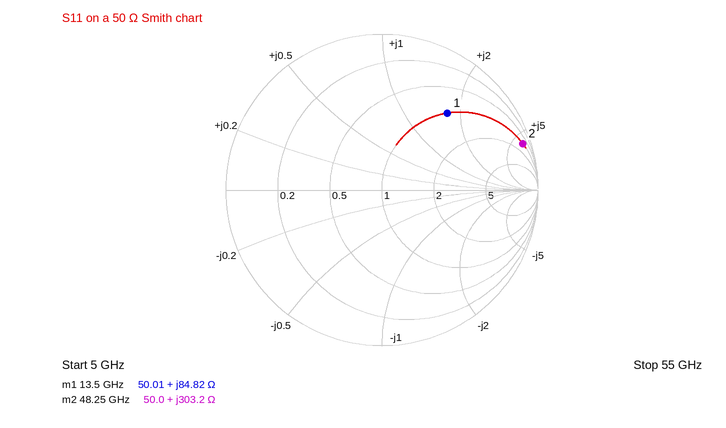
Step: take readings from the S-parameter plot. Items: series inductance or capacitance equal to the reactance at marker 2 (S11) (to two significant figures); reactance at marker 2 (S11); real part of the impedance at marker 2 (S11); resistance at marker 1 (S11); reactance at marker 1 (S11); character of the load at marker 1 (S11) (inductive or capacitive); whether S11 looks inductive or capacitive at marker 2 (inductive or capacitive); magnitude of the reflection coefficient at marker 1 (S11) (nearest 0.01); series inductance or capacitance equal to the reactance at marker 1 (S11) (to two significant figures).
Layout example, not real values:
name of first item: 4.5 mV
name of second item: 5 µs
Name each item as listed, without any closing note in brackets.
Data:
series inductance or capacitance equal to the reactance at marker 2 (S11): 1.00 nH
reactance at marker 2: +303.2 Ω
real part of the impedance at marker 2: 50.0 Ω
resistance at marker 1: 50.01 Ω
reactance at marker 1: +84.82 Ω
character of the load at marker 1 (S11): inductive
whether S11 looks inductive or capacitive at marker 2: inductive
magnitude of the reflection coefficient at marker 1 (S11): 0.65
series inductance or capacitance equal to the reactance at marker 1 (S11): 1.00 nH
